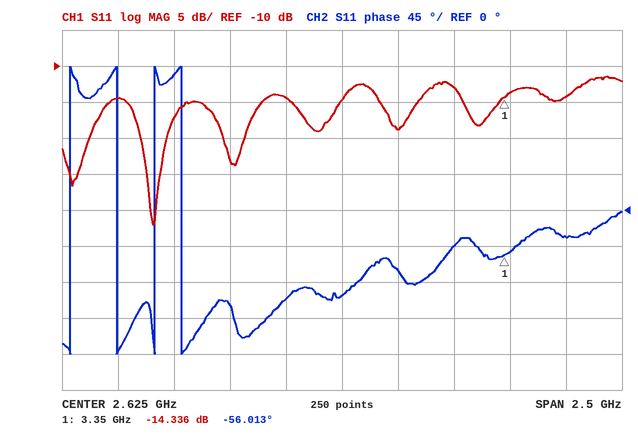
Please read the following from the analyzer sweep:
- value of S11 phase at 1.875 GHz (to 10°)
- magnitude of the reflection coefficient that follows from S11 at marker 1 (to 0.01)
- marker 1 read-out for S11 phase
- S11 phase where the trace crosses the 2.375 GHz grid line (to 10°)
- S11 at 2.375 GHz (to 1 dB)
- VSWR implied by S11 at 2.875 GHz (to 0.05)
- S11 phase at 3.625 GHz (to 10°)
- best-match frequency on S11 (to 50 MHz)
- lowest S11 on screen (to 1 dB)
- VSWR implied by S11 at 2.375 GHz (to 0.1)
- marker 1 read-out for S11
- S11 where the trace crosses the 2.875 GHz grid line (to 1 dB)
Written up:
170°
0.19
-56.013°
-110°
-14 dB
1.25
-30°
1.80 GHz
-32 dB
1.5
-14.336 dB
-19 dB
